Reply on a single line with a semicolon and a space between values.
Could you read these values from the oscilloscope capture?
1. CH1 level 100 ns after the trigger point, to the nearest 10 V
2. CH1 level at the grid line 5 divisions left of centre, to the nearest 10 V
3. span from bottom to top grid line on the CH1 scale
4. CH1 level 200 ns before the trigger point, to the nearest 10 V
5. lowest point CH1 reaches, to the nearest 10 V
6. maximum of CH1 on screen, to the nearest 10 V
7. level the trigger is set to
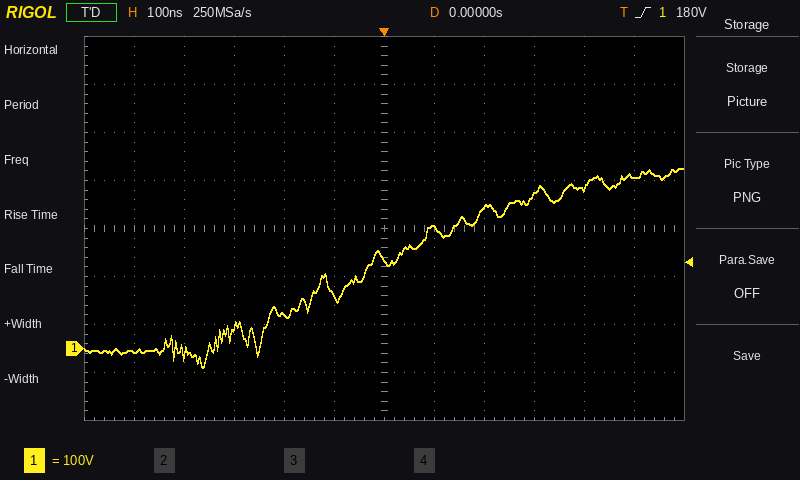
250 V; -10 V; 800 V; 70 V; -40 V; 380 V; 180 V
